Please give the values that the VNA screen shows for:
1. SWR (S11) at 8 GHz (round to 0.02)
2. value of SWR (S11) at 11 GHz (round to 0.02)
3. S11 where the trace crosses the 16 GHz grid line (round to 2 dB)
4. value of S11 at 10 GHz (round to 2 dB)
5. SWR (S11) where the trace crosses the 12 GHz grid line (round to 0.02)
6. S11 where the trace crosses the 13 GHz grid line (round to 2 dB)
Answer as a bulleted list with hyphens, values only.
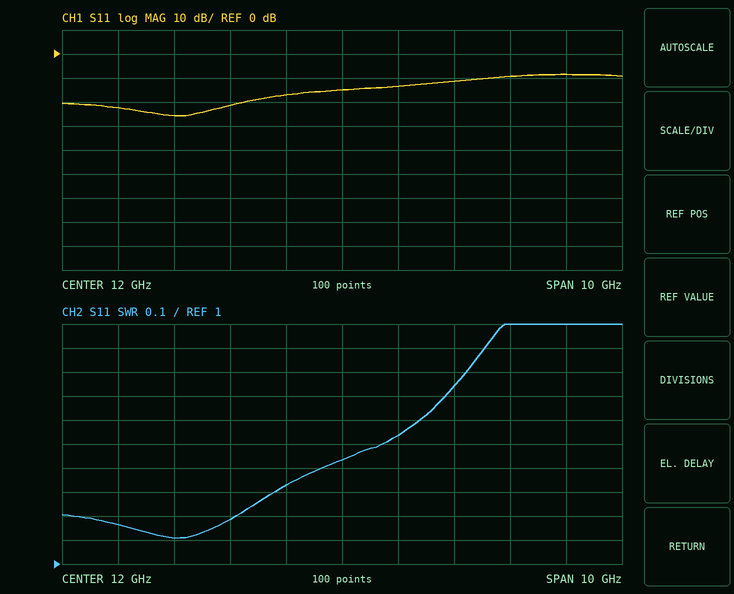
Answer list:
- 1.16
- 1.32
- -8 dB
- -22 dB
- 1.44
- -14 dB
